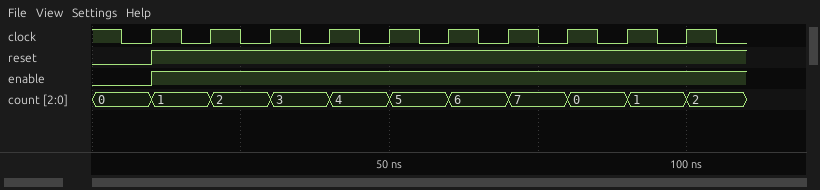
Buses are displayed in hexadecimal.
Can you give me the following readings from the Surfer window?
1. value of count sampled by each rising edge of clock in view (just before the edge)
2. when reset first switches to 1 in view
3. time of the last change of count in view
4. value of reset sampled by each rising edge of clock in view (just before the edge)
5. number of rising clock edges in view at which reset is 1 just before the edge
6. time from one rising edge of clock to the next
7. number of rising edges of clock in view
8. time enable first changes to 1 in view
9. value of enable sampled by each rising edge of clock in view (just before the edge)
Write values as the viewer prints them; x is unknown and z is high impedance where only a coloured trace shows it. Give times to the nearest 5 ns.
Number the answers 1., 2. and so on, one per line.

1. 0, 1, 2, 3, 4, 5, 6, 7, 0, 1
2. 10 ns
3. 100 ns
4. 0 1 1 1 1 1 1 1 1 1
5. 9
6. 10 ns
7. 10
8. 10 ns
9. 0 1 1 1 1 1 1 1 1 1
